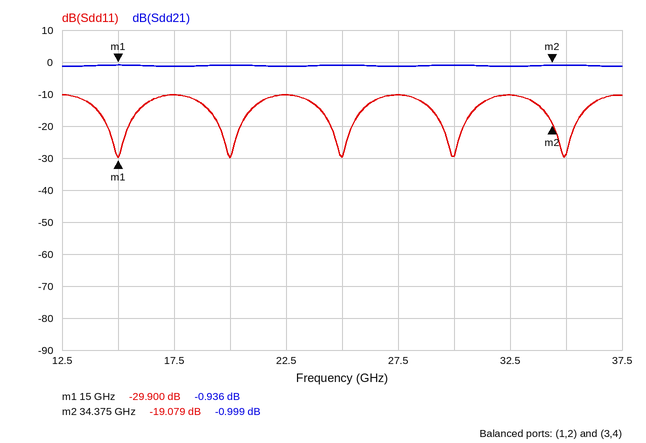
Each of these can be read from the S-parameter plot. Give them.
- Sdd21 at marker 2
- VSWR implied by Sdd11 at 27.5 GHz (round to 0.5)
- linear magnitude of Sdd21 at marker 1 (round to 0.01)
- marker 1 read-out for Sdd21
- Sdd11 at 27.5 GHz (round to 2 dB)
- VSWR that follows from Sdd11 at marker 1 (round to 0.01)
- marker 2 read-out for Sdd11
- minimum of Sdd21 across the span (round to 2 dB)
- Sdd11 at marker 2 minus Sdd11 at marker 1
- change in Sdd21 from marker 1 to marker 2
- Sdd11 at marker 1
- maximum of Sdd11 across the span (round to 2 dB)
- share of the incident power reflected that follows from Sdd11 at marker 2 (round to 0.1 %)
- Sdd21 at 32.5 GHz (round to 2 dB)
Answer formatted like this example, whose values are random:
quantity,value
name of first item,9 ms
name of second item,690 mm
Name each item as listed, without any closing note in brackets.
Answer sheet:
quantity,value
Sdd21 at marker 2,-0.999 dB
VSWR implied by Sdd11 at 27.5 GHz,2.0
linear magnitude of Sdd21 at marker 1,0.90
marker 1 read-out for Sdd21,-0.936 dB
Sdd11 at 27.5 GHz,-10 dB
VSWR that follows from Sdd11 at marker 1,1.07
marker 2 read-out for Sdd11,-19.079 dB
minimum of Sdd21 across the span,-2 dB
Sdd11 at marker 2 minus Sdd11 at marker 1,10.821 dB
change in Sdd21 from marker 1 to marker 2,-0.063 dB
Sdd11 at marker 1,-29.900 dB
maximum of Sdd11 across the span,-10 dB
share of the incident power reflected that follows from Sdd11 at marker 2,1.2 %
Sdd21 at 32.5 GHz,-2 dB
